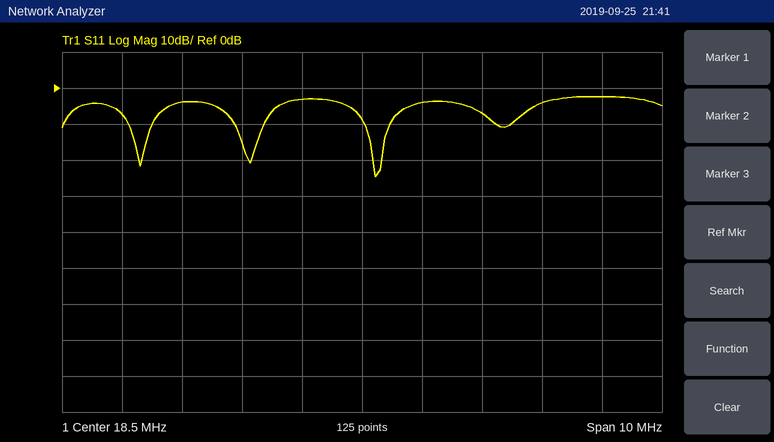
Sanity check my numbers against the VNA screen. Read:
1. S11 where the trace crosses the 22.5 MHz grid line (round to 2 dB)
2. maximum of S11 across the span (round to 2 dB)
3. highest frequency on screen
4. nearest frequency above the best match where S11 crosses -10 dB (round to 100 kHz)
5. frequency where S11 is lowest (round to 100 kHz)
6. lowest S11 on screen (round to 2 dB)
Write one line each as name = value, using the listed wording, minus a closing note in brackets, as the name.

S11 where the trace crosses the 22.5 MHz grid line = -2 dB
maximum of S11 across the span = -2 dB
highest frequency on screen = 23.5 MHz
nearest frequency above the best match where S11 crosses -10 dB = 19.0 MHz
frequency where S11 is lowest = 18.7 MHz
lowest S11 on screen = -24 dB
